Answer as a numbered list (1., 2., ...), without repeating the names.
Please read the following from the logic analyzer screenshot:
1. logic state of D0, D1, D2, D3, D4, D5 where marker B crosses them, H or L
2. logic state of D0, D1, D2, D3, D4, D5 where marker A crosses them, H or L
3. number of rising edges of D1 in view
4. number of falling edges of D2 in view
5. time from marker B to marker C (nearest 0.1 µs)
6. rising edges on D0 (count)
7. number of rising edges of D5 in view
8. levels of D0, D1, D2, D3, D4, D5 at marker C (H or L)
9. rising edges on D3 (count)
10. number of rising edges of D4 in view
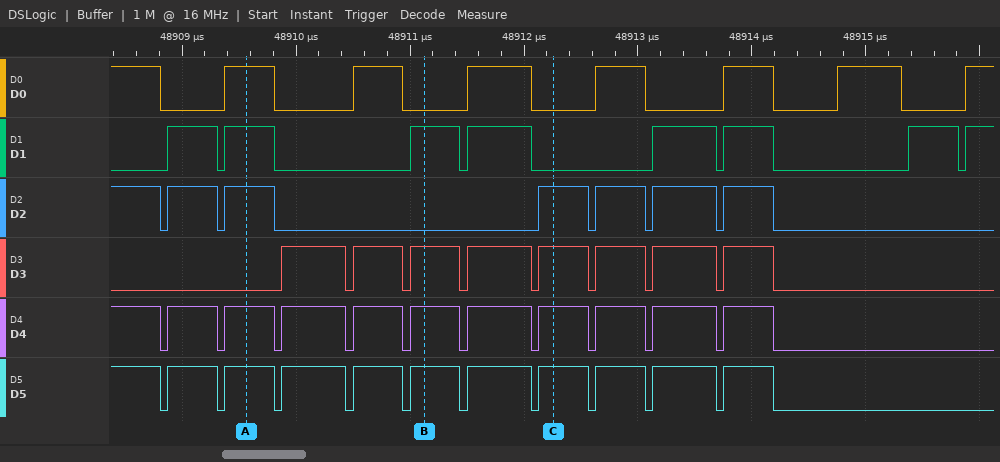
1. D0=L, D1=H, D2=L, D3=H, D4=H, D5=H
2. D0=H, D1=H, D2=H, D3=L, D4=H, D5=H
3. 8
4. 7
5. 1.1 µs
6. 7
7. 10
8. D0=L, D1=L, D2=H, D3=H, D4=H, D5=H
9. 8
10. 10
